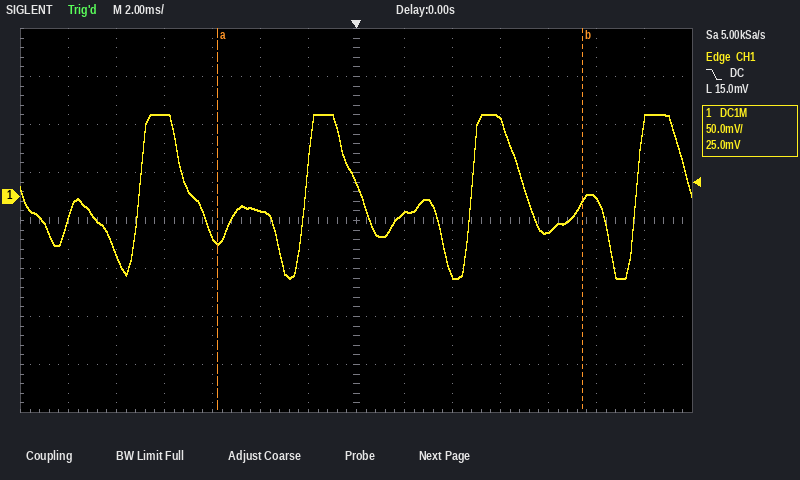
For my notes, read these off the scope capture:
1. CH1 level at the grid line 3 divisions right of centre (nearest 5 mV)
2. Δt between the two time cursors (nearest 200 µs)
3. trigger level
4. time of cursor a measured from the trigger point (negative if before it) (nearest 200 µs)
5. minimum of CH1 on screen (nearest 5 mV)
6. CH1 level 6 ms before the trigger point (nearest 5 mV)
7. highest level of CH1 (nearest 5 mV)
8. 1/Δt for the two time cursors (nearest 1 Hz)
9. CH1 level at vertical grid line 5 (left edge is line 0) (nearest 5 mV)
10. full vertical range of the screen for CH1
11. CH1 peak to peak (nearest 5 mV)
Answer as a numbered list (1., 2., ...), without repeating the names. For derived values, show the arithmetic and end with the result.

1. 80 mV
2. 15.2 ms
3. 15.0 mV
4. -5.8 ms
5. -85 mV
6. -40 mV
7. 85 mV
8. 1 / 15.2 ms ≈ 66 Hz
9. -15 mV
10. 400 mV
11. 85 mV − (-85 mV) = 170 mV
